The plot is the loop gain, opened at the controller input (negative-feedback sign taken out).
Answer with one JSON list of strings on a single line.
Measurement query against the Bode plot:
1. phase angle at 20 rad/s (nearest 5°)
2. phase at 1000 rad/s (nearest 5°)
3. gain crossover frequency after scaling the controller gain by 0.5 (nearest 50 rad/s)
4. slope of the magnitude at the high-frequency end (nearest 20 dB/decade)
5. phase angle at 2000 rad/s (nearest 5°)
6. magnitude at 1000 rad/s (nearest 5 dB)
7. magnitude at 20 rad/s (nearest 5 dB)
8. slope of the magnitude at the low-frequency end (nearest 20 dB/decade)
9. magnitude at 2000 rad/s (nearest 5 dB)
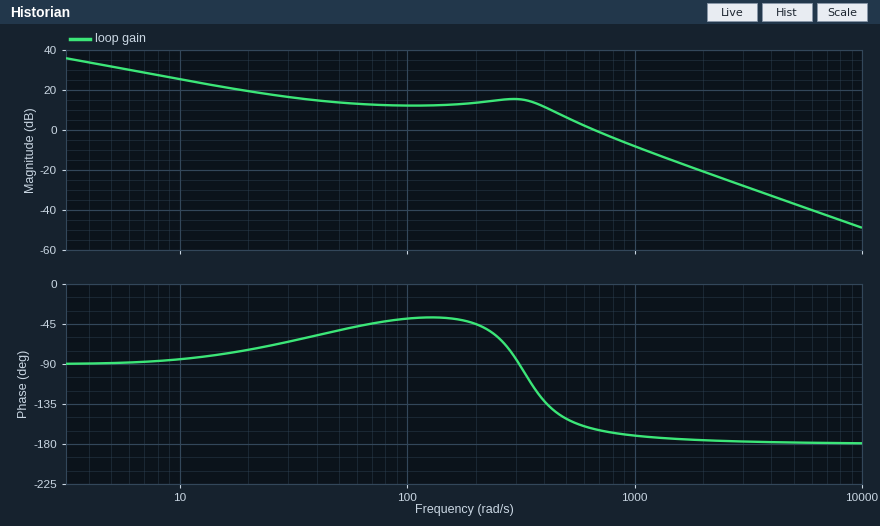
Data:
["-75°", "-170°", "500 rad/s", "-40 dB/decade", "-175°", "-10 dB", "20 dB", "-20 dB/decade", "-20 dB"]
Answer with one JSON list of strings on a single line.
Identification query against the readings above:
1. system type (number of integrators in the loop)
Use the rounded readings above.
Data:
["1"]
